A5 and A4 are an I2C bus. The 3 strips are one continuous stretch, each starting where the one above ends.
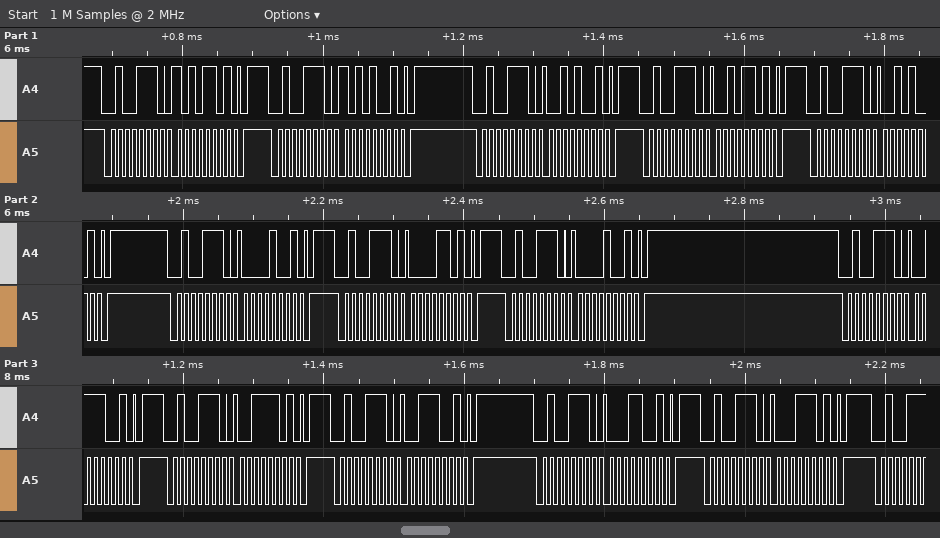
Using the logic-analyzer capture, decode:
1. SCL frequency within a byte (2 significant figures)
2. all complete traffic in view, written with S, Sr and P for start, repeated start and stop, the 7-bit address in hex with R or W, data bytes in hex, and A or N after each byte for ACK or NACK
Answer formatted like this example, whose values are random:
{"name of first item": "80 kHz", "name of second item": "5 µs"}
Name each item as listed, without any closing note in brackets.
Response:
{"SCL frequency within a byte": "100 kHz", "all complete traffic in view, written with S, Sr and P for start, repeated start and stop, the 7-bit address in hex with R or W, data bytes in hex, and A or N after each byte for ACK or NACK": "S 27W A AD A P S 27W A A9 A P S 27W A 29 A P S 27W A 2D A P S 27W A 29 A P S 27W A 09 A P S 27W A 0D A P S 27W A 09 A P S 27W A 39 A P S 27W A 3D A P S 27W A 39 A P S 27W A 19 A P S 27W A 1D A P"}
